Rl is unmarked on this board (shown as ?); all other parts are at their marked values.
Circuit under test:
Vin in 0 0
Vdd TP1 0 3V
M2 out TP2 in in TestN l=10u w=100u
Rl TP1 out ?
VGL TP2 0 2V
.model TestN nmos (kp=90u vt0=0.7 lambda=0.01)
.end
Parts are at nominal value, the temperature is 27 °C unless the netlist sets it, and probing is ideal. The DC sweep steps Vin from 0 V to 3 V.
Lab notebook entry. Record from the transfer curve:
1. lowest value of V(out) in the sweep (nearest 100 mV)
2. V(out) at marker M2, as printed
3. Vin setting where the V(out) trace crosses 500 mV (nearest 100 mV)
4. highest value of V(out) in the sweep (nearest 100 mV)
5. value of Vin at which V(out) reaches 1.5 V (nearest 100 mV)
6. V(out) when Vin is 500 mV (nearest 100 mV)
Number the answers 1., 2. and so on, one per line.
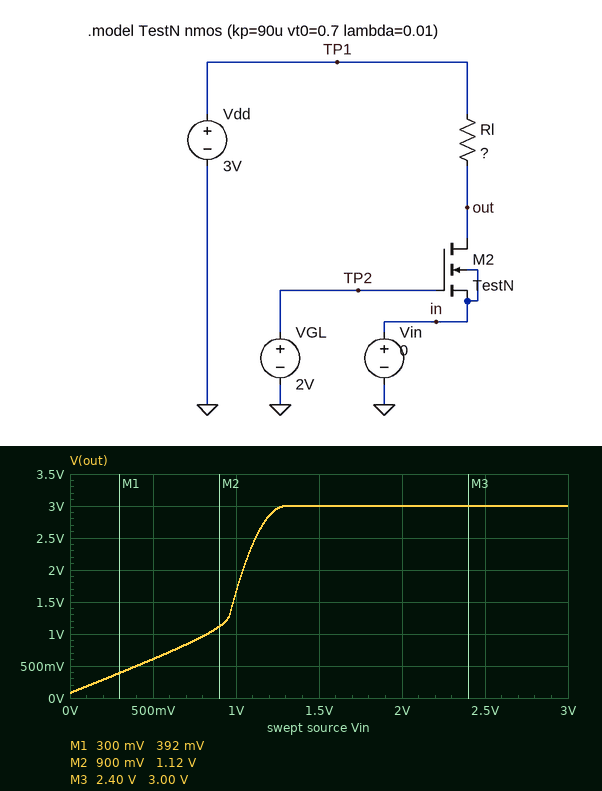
1. 100 mV
2. 1.12 V
3. 400 mV
4. 3.0 V
5. 1.0 V
6. 600 mV
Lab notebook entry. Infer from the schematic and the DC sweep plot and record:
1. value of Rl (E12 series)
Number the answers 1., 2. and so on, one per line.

1. 33 kΩ
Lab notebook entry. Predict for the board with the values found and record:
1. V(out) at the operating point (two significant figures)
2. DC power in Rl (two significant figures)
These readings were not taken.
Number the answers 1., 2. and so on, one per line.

1. 78 mV
2. 260 µW
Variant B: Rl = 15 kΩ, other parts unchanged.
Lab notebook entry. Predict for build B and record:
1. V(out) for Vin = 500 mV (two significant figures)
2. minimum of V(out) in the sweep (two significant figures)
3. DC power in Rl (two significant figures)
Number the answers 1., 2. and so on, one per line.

1. 750 mV
2. 170 mV
3. 530 µW
